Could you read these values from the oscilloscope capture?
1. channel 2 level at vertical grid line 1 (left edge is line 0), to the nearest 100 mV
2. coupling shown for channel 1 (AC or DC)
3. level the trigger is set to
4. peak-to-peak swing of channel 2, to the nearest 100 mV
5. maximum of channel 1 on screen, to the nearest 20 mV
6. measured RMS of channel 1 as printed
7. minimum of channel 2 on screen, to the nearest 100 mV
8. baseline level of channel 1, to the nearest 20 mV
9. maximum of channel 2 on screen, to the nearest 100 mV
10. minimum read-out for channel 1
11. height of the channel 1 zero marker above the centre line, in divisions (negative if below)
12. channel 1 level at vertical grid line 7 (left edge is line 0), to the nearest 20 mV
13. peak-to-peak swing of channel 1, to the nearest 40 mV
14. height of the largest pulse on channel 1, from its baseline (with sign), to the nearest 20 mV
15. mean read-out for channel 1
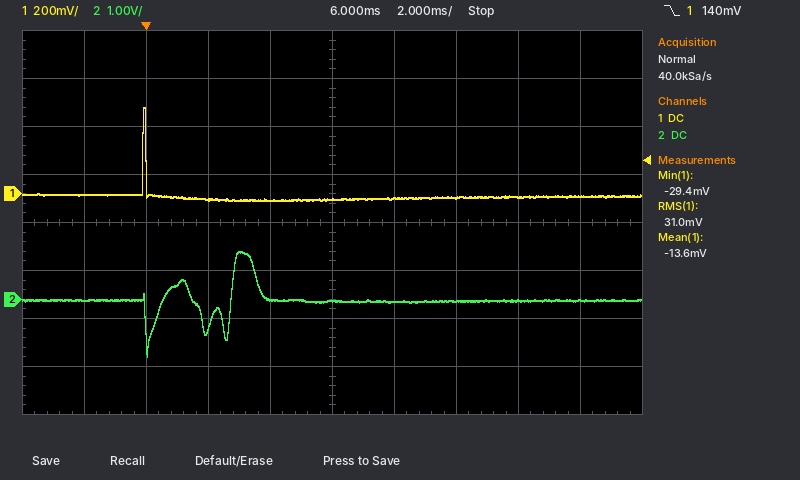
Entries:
0.0 V
DC
140 mV
2.2 V
360 mV
31.0 mV
-1.2 V
-20 mV
1.0 V
-29.4 mV
+0.6 div
-20 mV
400 mV
+380 mV
-13.6 mV
